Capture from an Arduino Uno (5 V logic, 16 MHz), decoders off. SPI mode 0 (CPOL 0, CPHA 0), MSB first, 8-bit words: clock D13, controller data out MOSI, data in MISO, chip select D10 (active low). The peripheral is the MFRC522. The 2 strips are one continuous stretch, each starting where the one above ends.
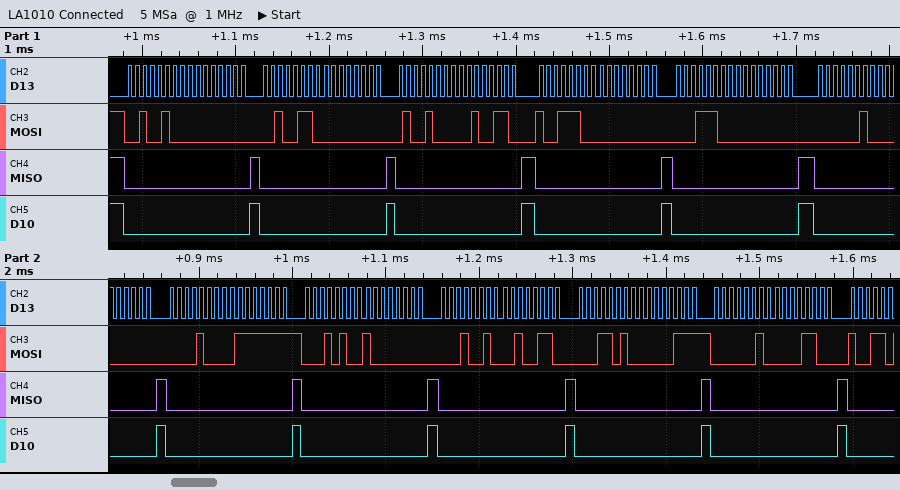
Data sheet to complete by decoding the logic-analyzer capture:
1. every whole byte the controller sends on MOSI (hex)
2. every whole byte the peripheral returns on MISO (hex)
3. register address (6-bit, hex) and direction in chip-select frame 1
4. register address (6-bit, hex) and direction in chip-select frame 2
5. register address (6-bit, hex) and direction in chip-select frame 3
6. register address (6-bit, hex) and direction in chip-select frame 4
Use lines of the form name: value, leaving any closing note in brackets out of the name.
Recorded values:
every whole byte the controller sends on MOSI: 24 00 26 00 48 26 9C 00 1C 00 02 00 08 7F 14 80 12 26 1A 07 02 0C
every whole byte the peripheral returns on MISO: 00 00 00 00 00 00 00 00 00 00 00 00 00 00 00 00 00 00 00 00 00 00
register address (6-bit, hex) and direction in chip-select frame 1: 0x12 write
register address (6-bit, hex) and direction in chip-select frame 2: 0x13 write
register address (6-bit, hex) and direction in chip-select frame 3: 0x24 write
register address (6-bit, hex) and direction in chip-select frame 4: 0x0E read
